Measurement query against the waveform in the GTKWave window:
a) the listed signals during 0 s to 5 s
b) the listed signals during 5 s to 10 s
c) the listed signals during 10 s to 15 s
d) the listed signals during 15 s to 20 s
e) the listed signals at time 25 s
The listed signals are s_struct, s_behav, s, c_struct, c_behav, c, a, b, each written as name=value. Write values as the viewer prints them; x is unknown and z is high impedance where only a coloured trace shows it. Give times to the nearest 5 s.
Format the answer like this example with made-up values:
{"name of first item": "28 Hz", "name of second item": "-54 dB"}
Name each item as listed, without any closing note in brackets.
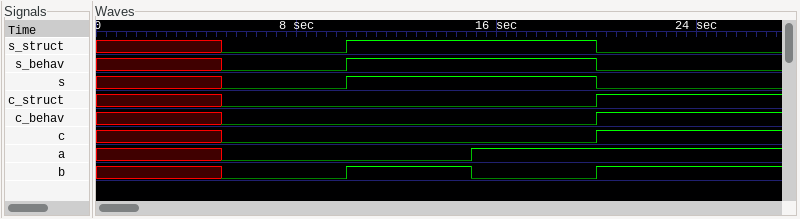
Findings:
{"the listed signals during 0 s to 5 s": "s_struct=x, s_behav=x, s=x, c_struct=x, c_behav=x, c=x, a=x, b=x", "the listed signals during 5 s to 10 s": "s_struct=0, s_behav=0, s=0, c_struct=0, c_behav=0, c=0, a=0, b=0", "the listed signals during 10 s to 15 s": "s_struct=1, s_behav=1, s=1, c_struct=0, c_behav=0, c=0, a=0, b=1", "the listed signals during 15 s to 20 s": "s_struct=1, s_behav=1, s=1, c_struct=0, c_behav=0, c=0, a=1, b=0", "the listed signals at time 25 s": "s_struct=0, s_behav=0, s=0, c_struct=1, c_behav=1, c=1, a=1, b=1"}
